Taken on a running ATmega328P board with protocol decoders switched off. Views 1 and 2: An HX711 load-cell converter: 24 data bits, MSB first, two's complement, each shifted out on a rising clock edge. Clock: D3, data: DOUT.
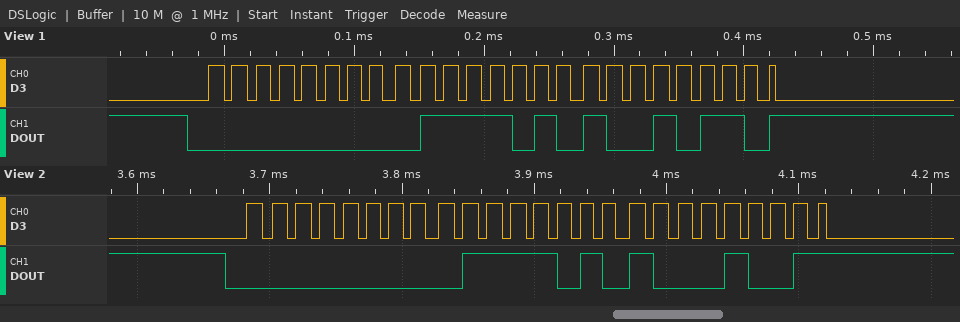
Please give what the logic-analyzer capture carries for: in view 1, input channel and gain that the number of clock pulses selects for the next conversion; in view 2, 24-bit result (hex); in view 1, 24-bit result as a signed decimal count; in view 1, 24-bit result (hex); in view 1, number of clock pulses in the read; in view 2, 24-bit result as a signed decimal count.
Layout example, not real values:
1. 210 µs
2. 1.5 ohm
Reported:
1. channel A, gain 128
2. 0x007A89
3. 31382
4. 0x007A96
5. 25
6. 31369
